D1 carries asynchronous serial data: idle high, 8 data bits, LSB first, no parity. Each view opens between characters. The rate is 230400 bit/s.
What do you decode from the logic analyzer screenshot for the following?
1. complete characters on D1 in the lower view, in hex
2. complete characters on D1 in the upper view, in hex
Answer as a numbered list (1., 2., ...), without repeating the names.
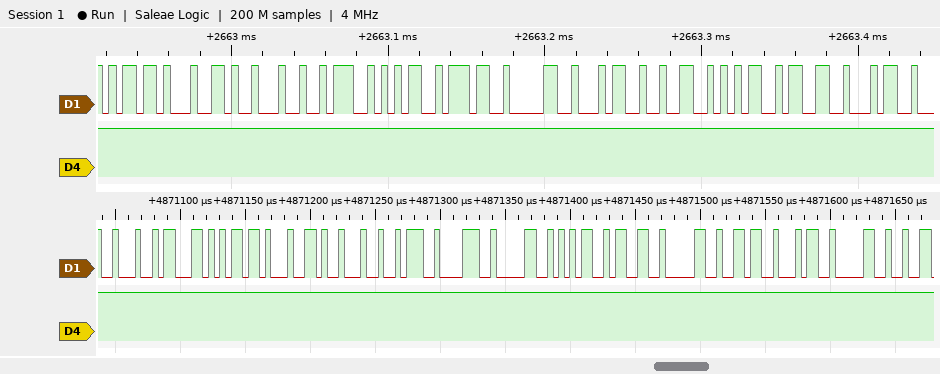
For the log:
1. 22, 63, 6D, 64, 22, 3A, 38, 30, 35, 33, 30, 36, 34, 30
2. 6D, 64, 22, 3A, 35, 37, 30, 34, 32, 35, 33, 34
